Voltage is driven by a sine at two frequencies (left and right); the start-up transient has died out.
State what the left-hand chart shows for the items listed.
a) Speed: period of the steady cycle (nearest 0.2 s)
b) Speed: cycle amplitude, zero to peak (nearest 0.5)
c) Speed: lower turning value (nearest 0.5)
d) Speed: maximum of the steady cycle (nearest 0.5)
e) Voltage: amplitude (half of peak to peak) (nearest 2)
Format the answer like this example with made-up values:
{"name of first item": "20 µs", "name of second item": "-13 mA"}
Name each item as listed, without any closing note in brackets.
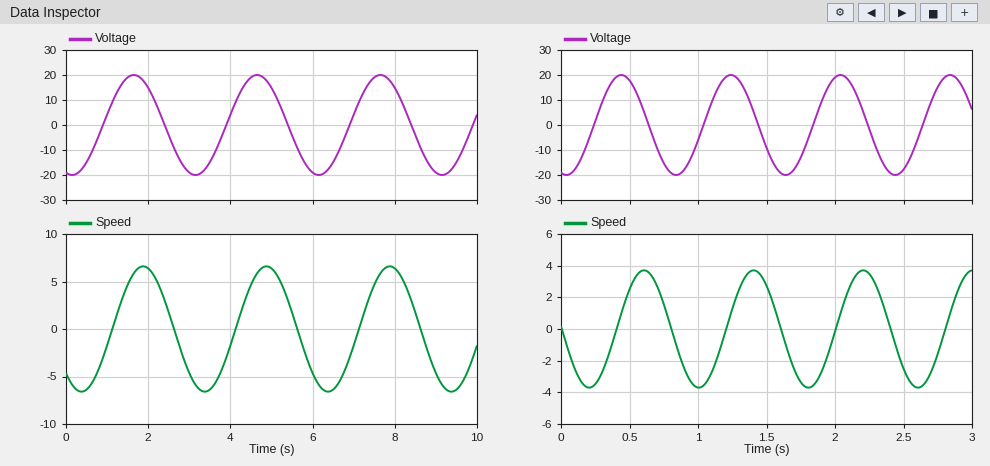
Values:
{"Speed: period of the steady cycle": "3.0 s", "Speed: cycle amplitude, zero to peak": "6.5", "Speed: lower turning value": "-6.5", "Speed: maximum of the steady cycle": "6.5", "Voltage: amplitude (half of peak to peak)": "20"}
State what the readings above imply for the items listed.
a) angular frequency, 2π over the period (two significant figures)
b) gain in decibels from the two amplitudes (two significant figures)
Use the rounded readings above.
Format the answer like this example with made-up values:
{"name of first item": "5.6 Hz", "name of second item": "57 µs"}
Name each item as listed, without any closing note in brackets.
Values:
{"angular frequency, 2π over the period": "2.1 rad/s", "gain in decibels from the two amplitudes": "-9.8 dB"}
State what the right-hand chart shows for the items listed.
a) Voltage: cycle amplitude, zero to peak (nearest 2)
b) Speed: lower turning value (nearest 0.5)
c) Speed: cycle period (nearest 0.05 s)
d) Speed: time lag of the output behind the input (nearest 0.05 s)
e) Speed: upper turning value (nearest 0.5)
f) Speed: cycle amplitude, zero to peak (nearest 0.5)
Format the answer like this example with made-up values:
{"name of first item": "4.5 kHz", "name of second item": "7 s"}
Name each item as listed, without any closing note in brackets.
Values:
{"Voltage: cycle amplitude, zero to peak": "20", "Speed: lower turning value": "-3.5", "Speed: cycle period": "0.80 s", "Speed: time lag of the output behind the input": "0.15 s", "Speed: upper turning value": "3.5", "Speed: cycle amplitude, zero to peak": "3.5"}
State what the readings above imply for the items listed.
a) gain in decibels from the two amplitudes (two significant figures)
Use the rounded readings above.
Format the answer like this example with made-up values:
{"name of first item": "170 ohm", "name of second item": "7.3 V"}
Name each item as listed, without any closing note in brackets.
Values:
{"gain in decibels from the two amplitudes": "-15 dB"}
